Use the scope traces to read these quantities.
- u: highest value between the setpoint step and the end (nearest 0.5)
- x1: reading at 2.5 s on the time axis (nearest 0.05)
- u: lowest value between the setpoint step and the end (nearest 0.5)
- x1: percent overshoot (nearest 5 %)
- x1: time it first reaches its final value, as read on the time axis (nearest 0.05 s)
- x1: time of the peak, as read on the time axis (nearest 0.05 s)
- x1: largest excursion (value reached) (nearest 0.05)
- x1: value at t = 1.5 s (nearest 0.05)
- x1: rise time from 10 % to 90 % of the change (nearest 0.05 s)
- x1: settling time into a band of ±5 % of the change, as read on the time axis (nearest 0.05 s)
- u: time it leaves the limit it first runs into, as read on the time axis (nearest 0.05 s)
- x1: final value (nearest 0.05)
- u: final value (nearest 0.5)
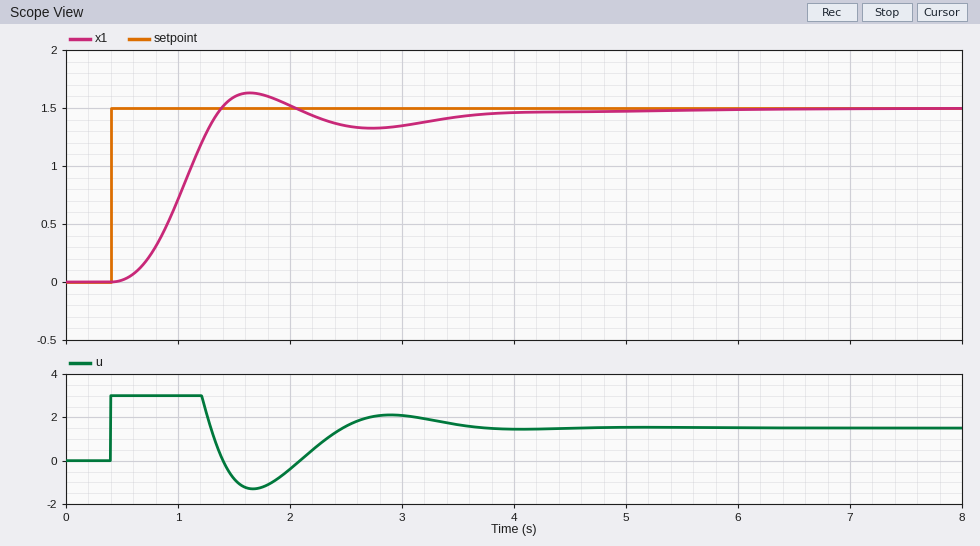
3.0
1.35
-1.5
10 %
1.40 s
1.65 s
1.65
1.60
0.60 s
3.50 s
1.20 s
1.50
1.5
